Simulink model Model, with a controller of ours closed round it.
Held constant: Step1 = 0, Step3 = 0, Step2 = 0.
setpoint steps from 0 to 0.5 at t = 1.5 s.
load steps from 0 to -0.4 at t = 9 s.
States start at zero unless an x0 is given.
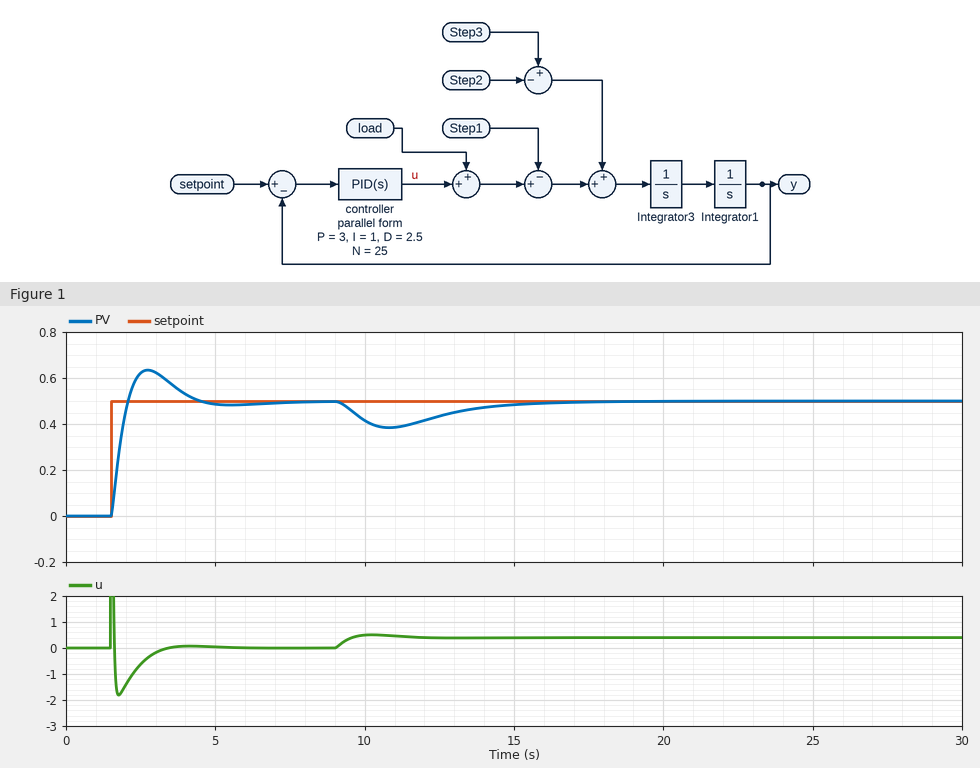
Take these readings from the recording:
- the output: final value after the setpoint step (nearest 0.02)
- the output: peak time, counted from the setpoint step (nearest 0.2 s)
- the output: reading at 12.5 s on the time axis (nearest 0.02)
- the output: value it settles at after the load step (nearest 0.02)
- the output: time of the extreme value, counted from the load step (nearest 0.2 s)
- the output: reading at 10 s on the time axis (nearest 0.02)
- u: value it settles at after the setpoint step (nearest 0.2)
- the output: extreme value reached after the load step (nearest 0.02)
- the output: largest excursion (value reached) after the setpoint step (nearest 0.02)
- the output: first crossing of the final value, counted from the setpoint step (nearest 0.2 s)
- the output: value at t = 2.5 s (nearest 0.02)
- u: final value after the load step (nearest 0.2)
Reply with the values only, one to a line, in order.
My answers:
0.50
1.2 s
0.44
0.50
1.8 s
0.42
0.0
0.38
0.64
0.6 s
0.62
0.4
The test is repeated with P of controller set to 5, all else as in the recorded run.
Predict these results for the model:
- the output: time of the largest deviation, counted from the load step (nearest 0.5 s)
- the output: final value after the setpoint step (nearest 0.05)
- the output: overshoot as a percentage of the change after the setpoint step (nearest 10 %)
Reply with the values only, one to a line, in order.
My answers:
1.5 s
0.50
30 %
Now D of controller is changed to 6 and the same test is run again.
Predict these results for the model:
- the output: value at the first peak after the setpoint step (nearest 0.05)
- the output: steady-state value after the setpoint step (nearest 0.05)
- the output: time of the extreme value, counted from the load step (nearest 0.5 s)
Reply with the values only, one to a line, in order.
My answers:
0.55
0.50
3.0 s
